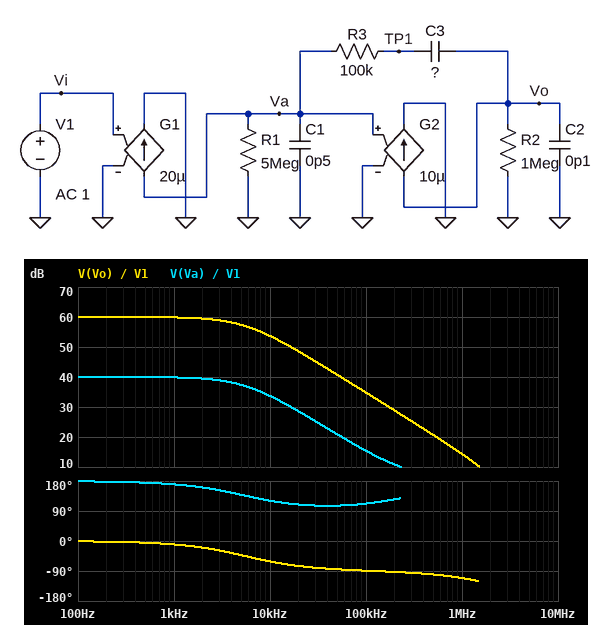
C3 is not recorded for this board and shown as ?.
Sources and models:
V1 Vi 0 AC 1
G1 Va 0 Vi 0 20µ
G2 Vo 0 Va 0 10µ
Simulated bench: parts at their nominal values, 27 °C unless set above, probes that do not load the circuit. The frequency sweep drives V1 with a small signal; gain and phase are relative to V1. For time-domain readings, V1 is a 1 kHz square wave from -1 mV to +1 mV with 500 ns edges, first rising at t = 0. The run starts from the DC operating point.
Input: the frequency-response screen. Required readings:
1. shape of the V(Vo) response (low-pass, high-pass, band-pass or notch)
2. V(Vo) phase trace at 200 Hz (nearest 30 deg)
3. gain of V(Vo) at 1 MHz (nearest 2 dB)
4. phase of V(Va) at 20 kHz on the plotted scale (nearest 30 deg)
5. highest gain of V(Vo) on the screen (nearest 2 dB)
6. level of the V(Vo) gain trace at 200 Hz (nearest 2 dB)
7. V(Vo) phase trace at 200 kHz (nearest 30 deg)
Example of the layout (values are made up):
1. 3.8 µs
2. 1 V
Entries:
1. low-pass
2. 0 deg
3. 14 dB
4. 120 deg
5. 60 dB
6. 60 dB
7. -90 deg
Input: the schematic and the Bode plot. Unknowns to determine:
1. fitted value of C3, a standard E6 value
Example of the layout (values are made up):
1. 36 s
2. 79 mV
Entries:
1. 470 fF
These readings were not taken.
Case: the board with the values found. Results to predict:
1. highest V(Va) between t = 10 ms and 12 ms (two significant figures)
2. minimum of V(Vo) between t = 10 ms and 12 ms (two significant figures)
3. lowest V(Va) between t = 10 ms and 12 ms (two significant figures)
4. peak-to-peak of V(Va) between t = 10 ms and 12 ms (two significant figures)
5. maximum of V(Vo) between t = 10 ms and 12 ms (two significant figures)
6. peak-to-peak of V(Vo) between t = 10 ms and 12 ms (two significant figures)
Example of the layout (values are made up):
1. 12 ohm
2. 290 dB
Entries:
1. 100 mV
2. -1.0 V
3. -100 mV
4. 200 mV
5. 1.0 V
6. 2.0 V
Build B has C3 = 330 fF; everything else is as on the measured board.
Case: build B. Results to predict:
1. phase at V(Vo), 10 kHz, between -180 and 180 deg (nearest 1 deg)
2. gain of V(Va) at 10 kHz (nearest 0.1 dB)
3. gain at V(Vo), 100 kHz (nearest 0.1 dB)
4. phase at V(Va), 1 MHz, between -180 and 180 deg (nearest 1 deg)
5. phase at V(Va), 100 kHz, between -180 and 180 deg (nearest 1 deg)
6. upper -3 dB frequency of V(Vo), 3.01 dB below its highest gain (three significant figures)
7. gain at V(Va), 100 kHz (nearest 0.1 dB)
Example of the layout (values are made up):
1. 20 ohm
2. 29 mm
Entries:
1. -53 deg
2. 35.6 dB
3. 37.5 dB
4. 142 deg
5. 108 deg
6. 7.56 kHz
7. 17.9 dB
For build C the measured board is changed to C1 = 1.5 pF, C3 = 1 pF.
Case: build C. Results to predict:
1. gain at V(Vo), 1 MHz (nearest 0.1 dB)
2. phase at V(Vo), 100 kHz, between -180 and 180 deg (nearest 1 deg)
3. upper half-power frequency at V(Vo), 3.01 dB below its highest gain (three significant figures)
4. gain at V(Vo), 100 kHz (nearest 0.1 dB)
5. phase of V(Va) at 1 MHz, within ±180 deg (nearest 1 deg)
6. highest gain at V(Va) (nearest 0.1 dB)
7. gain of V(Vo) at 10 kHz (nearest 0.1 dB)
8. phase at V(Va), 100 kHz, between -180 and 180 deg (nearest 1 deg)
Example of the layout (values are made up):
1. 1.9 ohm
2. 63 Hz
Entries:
1. 5.4 dB
2. -94 deg
3. 2.50 kHz
4. 27.9 dB
5. 131 deg
6. 40.0 dB
7. 47.7 dB
8. 123 deg
